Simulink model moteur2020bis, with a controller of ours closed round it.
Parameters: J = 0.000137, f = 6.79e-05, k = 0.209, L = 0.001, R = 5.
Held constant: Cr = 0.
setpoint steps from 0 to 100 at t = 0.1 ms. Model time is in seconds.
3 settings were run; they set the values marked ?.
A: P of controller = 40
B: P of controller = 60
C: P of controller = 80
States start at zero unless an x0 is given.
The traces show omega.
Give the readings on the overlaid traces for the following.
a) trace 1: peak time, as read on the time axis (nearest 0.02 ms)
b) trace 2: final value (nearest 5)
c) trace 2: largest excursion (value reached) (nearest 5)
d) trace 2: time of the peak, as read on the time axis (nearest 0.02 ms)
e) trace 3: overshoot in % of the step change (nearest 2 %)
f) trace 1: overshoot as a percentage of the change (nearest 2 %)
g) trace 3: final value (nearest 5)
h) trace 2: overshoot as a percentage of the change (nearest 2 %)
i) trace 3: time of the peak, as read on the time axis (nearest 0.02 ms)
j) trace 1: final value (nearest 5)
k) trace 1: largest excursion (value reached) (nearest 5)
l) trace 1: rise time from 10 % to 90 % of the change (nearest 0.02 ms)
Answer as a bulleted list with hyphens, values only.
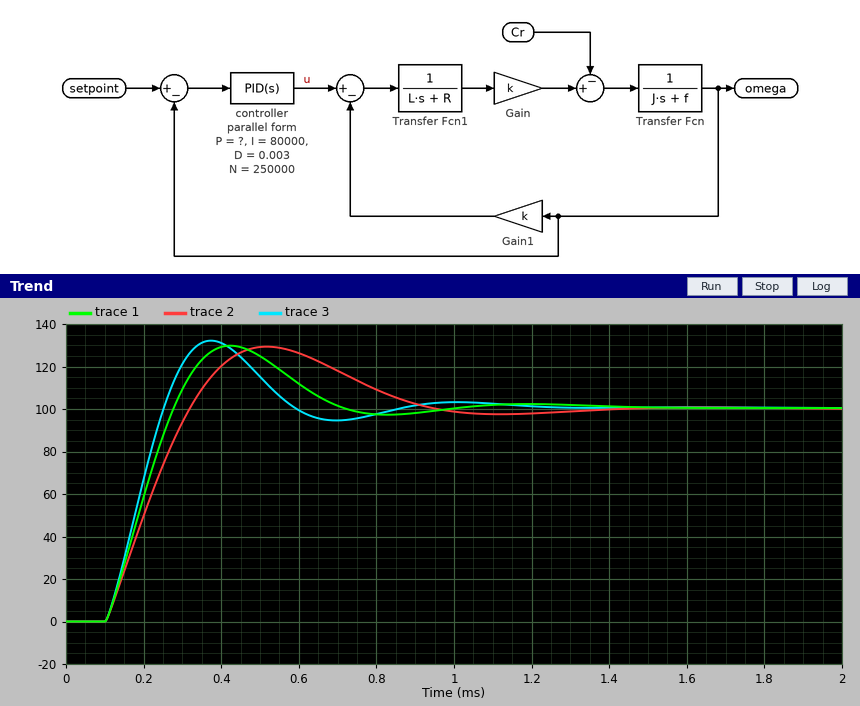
- 0.42 ms
- 100
- 130
- 0.52 ms
- 32 %
- 30 %
- 100
- 30 %
- 0.38 ms
- 100
- 130
- 0.14 ms
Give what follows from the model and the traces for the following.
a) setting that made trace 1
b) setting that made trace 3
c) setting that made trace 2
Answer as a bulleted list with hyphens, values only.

- B
- C
- A
